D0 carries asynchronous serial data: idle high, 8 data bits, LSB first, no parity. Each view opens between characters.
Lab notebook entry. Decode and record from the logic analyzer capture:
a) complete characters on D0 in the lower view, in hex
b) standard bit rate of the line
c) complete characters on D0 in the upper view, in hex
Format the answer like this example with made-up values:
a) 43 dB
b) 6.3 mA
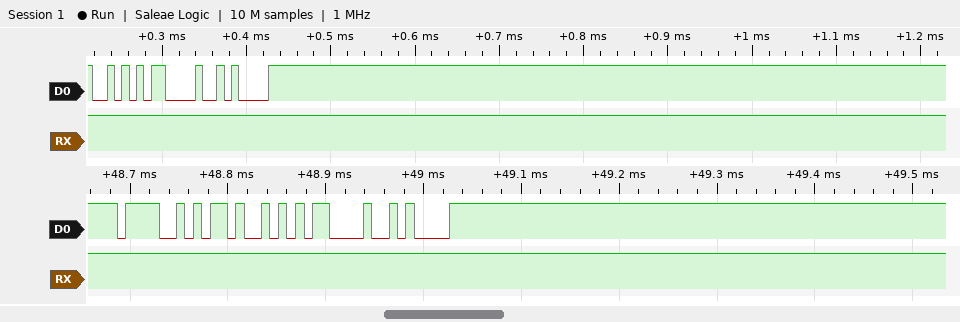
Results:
a) 4F, 4B, 0D, 0A
b) 115200 baud
c) AA, 48, F8
